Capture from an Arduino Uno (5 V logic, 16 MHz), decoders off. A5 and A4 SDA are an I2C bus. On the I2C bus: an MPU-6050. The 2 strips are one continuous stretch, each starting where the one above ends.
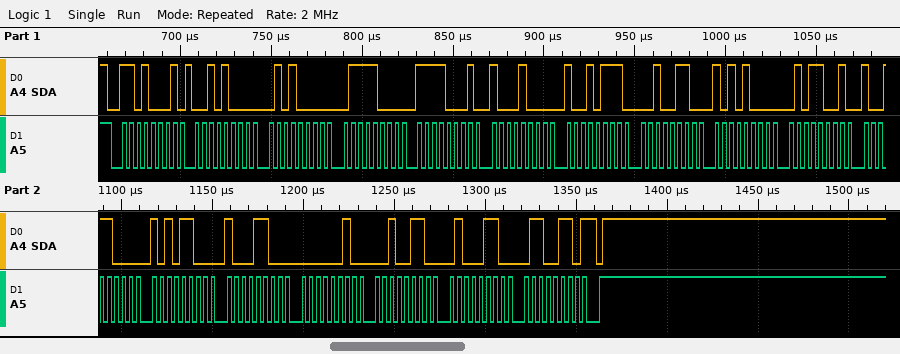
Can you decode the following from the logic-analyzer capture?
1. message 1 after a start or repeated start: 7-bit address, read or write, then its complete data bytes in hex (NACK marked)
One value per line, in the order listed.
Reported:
0x68 read: 28 50 78 F1 88 97 26 A8 59 98 AC 8C 02 26 46 66 NACK
